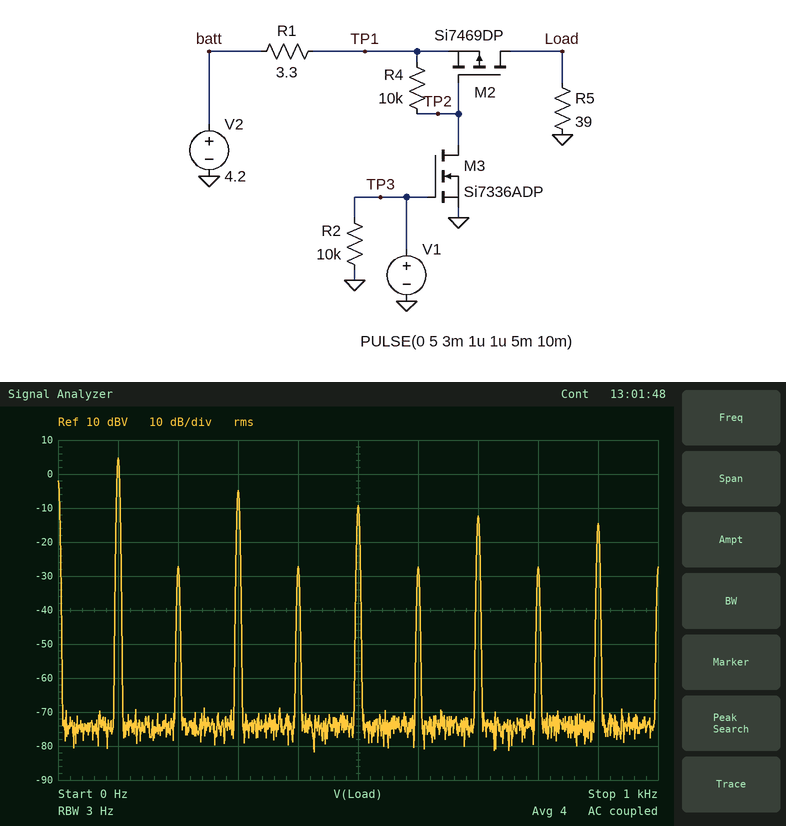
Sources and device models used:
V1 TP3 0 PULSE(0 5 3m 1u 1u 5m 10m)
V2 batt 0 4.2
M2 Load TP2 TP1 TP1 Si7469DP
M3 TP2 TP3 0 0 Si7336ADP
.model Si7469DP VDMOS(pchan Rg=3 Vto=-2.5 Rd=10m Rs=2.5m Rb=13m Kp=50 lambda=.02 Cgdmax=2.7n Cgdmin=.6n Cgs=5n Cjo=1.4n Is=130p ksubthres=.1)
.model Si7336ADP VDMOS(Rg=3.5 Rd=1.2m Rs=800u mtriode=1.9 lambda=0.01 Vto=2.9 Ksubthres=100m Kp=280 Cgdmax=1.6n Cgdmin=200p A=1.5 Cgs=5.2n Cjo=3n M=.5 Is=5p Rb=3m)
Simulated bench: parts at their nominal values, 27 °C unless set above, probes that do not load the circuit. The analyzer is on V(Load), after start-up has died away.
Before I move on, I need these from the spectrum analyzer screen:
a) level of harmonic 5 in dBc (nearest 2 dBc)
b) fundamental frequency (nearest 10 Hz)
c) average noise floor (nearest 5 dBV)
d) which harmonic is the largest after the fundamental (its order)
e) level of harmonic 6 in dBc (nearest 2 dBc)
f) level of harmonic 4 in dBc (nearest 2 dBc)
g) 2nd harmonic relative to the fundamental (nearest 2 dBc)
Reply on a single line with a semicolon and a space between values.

-14 dBc; 100 Hz; -75 dBV; 3; -32 dBc; -32 dBc; -32 dBc
